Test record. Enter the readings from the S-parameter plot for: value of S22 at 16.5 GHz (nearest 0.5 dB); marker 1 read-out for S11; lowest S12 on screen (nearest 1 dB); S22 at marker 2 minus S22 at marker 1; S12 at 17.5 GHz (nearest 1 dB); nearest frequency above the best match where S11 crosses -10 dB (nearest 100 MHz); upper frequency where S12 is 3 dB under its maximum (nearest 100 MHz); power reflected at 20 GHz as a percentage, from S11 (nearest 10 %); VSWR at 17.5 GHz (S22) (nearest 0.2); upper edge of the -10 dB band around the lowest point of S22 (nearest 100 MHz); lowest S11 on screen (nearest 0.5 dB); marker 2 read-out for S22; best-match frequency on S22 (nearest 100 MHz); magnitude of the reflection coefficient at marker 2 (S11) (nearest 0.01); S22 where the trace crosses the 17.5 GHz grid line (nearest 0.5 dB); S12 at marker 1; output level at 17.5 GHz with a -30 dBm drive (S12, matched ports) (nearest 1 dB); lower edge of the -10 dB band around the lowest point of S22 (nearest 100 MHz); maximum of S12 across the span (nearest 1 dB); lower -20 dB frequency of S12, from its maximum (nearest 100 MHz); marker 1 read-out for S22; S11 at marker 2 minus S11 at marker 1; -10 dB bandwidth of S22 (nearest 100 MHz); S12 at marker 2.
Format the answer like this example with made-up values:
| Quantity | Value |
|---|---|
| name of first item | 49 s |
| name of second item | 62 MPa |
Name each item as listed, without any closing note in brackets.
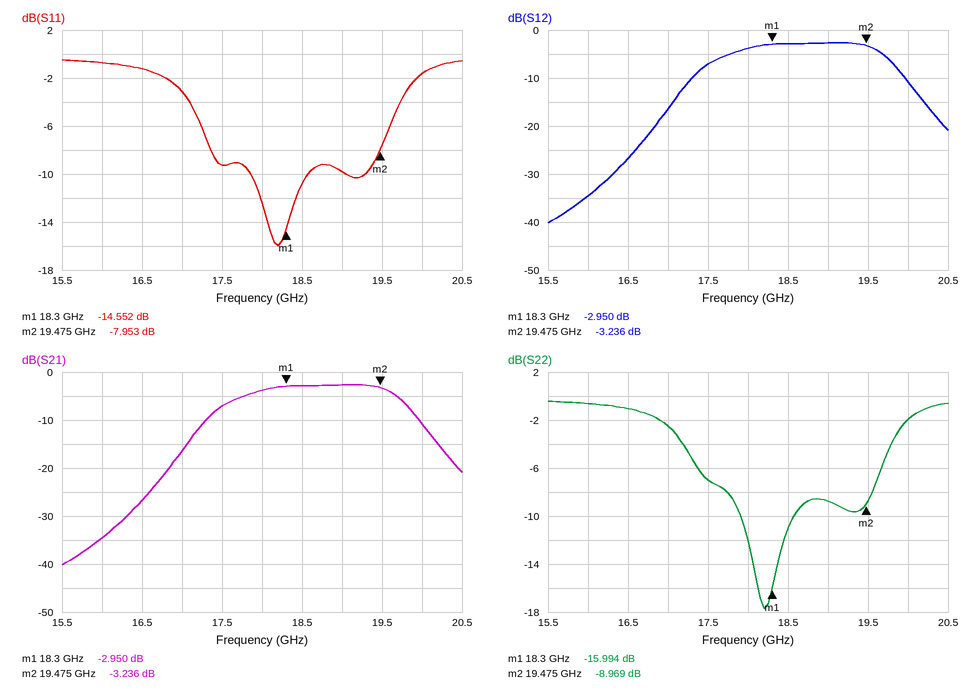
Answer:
| Quantity | Value |
|---|---|
| value of S22 at 16.5 GHz | -1.0 dB |
| marker 1 read-out for S11 | -14.552 dB |
| lowest S12 on screen | -40 dB |
| S22 at marker 2 minus S22 at marker 1 | 7.025 dB |
| S12 at 17.5 GHz | -7 dB |
| nearest frequency above the best match where S11 crosses -10 dB | 18.6 GHz |
| upper frequency where S12 is 3 dB under its maximum | 19.7 GHz |
| power reflected at 20 GHz as a percentage, from S11 | 70 % |
| VSWR at 17.5 GHz (S22) | 2.6 |
| upper edge of the -10 dB band around the lowest point of S22 | 18.6 GHz |
| lowest S11 on screen | -16.0 dB |
| marker 2 read-out for S22 | -8.969 dB |
| best-match frequency on S22 | 18.2 GHz |
| magnitude of the reflection coefficient at marker 2 (S11) | 0.40 |
| S22 where the trace crosses the 17.5 GHz grid line | -7.0 dB |
| S12 at marker 1 | -2.950 dB |
| output level at 17.5 GHz with a -30 dBm drive (S12, matched ports) | -37 dBm |
| lower edge of the -10 dB band around the lowest point of S22 | 17.9 GHz |
| maximum of S12 across the span | -3 dB |
| lower -20 dB frequency of S12, from its maximum | 16.7 GHz |
| marker 1 read-out for S22 | -15.994 dB |
| S11 at marker 2 minus S11 at marker 1 | 6.599 dB |
| -10 dB bandwidth of S22 | 700 MHz |
| S12 at marker 2 | -3.236 dB |
